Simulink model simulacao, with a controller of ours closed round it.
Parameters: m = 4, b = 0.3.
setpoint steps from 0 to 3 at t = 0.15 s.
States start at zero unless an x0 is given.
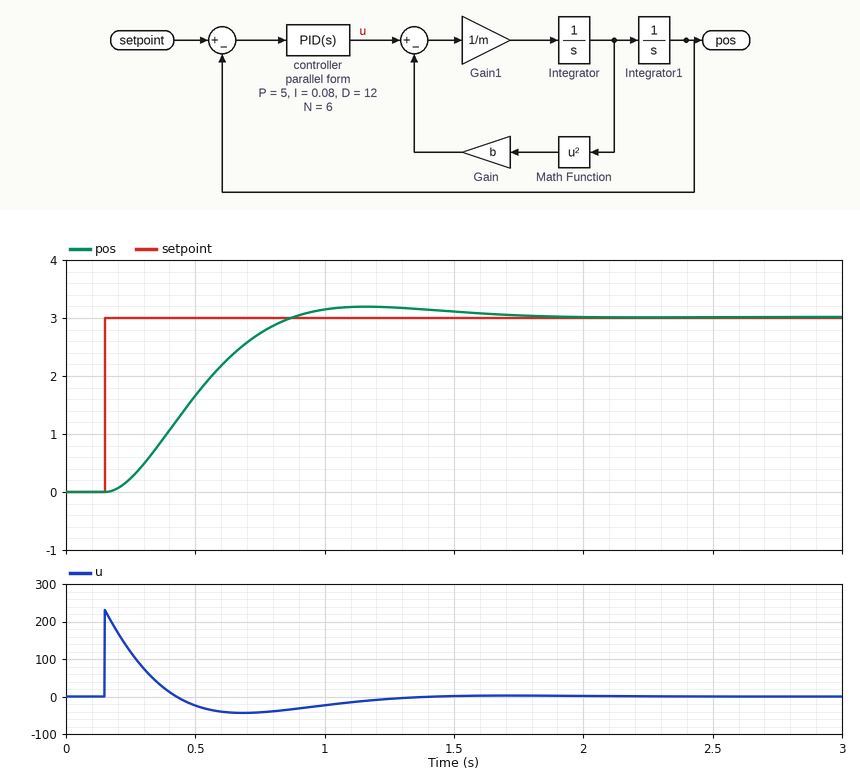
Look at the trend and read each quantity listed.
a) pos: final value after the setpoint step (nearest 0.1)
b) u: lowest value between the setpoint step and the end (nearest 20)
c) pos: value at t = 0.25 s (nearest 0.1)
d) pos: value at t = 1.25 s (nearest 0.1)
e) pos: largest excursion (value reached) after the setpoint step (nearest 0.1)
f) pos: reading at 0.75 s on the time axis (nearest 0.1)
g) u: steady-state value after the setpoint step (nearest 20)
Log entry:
3.0
-40
0.2
3.2
3.2
2.7
0
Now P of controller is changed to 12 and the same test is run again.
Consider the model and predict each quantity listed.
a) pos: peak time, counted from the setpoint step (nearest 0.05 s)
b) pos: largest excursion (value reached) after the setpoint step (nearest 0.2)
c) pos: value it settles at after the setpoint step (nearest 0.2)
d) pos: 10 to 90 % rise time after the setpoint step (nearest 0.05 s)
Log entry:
0.90 s
3.6
3.0
0.40 s
